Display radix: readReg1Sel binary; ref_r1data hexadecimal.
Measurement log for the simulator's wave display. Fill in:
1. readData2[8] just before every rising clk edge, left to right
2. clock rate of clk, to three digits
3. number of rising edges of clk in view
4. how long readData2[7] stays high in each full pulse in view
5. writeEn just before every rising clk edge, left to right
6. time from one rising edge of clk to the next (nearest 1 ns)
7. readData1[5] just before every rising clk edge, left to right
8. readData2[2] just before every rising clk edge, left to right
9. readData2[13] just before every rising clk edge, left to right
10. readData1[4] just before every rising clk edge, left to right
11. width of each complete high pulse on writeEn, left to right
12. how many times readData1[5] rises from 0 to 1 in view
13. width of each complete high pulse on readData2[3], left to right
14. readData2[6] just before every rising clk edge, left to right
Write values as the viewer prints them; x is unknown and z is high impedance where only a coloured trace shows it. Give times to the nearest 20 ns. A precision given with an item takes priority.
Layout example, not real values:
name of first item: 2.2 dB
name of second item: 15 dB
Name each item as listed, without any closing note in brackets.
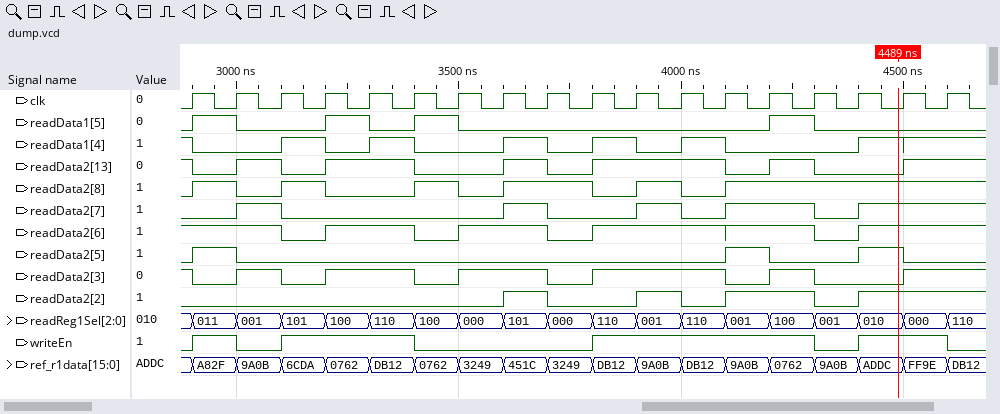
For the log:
readData2[8] just before every rising clk edge, left to right: 0 1 0 1 0 0 1 0 1 1 0 1 0 1 1 1 1 1
clock rate of clk, to three digits: 10.0 MHz
number of rising edges of clk in view: 18
how long readData2[7] stays high in each full pulse in view: 100 ns, 100 ns, 100 ns, 200 ns
writeEn just before every rising clk edge, left to right: 0 1 0 1 1 1 0 0 0 0 1 1 1 1 1 0 1 1
time from one rising edge of clk to the next: 100 ns
readData1[5] just before every rising clk edge, left to right: 0 1 0 0 1 0 1 0 0 0 0 0 0 0 1 0 0 0
readData2[2] just before every rising clk edge, left to right: 0 0 0 0 0 0 0 0 1 0 0 1 0 1 1 0 1 1
readData2[13] just before every rising clk edge, left to right: 1 0 1 0 1 1 0 0 1 0 1 1 1 0 1 0 0 1
readData1[4] just before every rising clk edge, left to right: 1 0 0 1 0 1 0 0 1 0 1 0 1 0 0 0 1 1
width of each complete high pulse on writeEn, left to right: 100 ns, 300 ns, 500 ns, 200 ns
how many times readData1[5] rises from 0 to 1 in view: 4
width of each complete high pulse on readData2[3], left to right: 100 ns, 200 ns, 200 ns, 300 ns, 100 ns
readData2[6] just before every rising clk edge, left to right: 1 1 1 0 1 1 0 1 1 0 1 1 1 1 1 0 1 1
